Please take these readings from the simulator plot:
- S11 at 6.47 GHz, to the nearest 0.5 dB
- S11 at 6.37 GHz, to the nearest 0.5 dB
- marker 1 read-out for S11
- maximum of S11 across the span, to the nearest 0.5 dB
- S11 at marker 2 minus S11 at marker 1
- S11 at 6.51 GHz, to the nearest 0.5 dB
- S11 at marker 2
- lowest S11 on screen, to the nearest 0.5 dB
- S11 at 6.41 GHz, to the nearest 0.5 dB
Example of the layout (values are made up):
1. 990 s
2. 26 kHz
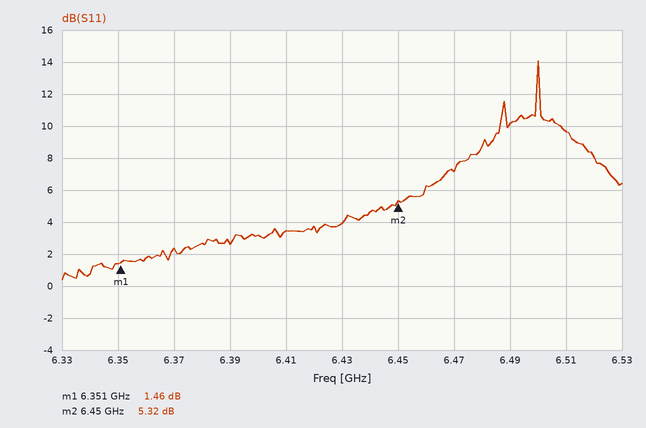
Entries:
1. 7.0 dB
2. 2.5 dB
3. 1.46 dB
4. 14.0 dB
5. 3.86 dB
6. 9.5 dB
7. 5.32 dB
8. 0.5 dB
9. 3.5 dB
